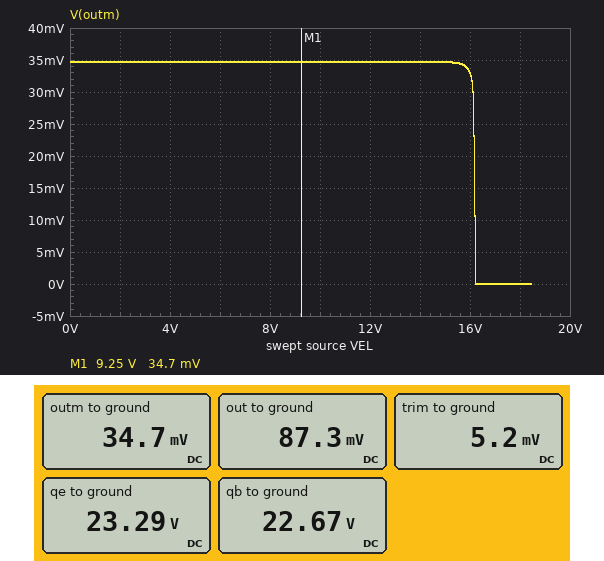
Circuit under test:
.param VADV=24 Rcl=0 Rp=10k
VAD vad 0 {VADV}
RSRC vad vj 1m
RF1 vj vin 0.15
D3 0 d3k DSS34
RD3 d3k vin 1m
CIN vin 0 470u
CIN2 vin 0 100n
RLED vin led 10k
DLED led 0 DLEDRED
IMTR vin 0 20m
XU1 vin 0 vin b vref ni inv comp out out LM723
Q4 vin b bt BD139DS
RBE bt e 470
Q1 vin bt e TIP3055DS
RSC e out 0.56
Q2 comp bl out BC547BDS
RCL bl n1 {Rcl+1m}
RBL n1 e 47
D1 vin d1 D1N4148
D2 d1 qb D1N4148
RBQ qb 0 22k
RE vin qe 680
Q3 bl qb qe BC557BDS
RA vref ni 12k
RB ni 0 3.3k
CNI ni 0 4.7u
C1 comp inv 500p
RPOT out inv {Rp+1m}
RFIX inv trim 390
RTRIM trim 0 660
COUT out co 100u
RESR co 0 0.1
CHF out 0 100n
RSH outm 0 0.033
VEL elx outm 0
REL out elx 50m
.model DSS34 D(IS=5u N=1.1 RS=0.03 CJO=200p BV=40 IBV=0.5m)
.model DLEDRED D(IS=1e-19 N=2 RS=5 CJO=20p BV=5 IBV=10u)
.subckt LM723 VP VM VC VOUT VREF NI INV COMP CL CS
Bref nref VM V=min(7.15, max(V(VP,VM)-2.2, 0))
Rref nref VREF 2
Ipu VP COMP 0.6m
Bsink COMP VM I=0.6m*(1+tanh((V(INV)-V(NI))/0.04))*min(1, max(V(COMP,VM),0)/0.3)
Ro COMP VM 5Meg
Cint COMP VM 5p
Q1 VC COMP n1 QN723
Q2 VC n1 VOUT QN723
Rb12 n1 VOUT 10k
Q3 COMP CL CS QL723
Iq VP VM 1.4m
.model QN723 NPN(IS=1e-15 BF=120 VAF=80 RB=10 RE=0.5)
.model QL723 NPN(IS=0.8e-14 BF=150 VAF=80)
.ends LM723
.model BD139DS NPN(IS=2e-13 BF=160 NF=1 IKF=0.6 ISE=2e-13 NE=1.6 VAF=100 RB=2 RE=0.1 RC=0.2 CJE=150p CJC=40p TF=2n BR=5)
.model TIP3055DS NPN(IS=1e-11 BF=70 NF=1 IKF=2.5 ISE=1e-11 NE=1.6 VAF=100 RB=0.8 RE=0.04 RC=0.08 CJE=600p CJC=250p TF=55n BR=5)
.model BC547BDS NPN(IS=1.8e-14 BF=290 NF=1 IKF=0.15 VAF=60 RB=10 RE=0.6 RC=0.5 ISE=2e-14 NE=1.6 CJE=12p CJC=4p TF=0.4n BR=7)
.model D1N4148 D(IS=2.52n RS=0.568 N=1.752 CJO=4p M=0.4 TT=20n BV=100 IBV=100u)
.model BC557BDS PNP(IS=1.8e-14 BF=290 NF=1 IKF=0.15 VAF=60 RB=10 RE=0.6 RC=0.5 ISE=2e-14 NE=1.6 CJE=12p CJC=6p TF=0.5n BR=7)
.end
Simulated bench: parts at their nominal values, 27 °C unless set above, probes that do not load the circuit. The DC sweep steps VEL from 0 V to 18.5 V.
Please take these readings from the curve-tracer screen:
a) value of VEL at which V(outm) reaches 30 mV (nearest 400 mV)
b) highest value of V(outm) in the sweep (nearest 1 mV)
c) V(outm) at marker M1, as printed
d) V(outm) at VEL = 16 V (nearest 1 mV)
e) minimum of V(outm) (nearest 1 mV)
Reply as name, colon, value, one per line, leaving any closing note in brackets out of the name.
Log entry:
value of VEL at which V(outm) reaches 30 mV: 16.0 V
highest value of V(outm) in the sweep: 35 mV
V(outm) at marker M1, as printed: 34.7 mV
V(outm) at VEL = 16 V: 33 mV
minimum of V(outm): 0 V
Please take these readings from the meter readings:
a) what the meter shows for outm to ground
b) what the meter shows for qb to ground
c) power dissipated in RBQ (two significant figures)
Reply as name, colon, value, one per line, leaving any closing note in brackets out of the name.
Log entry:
what the meter shows for outm to ground: 34.7 mV
what the meter shows for qb to ground: 22.67 V
power dissipated in RBQ: 23 mW
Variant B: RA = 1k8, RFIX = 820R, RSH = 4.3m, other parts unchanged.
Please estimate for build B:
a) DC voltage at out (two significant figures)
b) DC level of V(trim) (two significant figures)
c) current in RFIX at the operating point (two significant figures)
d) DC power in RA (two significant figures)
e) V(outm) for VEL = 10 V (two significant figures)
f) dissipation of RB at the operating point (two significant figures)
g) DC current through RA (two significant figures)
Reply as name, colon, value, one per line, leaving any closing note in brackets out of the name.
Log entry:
DC voltage at out: 57 mV
DC level of V(trim): 3.3 mV
current in RFIX at the operating point: 5.0 µA
DC power in RA: 3.5 mW
V(outm) for VEL = 10 V: 4.5 mV
dissipation of RB at the operating point: 6.5 mW
DC current through RA: 1.4 mA
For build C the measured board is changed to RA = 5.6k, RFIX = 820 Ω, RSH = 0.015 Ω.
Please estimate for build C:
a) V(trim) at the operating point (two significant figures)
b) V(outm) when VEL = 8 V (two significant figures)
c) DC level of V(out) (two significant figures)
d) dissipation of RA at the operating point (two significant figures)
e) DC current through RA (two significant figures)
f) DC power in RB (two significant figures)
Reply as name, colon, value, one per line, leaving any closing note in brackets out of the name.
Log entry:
V(trim) at the operating point: 3.9 mV
V(outm) when VEL = 8 V: 16 mV
DC level of V(out): 68 mV
dissipation of RA at the operating point: 3.6 mW
DC current through RA: 800 µA
DC power in RB: 2.1 mW
